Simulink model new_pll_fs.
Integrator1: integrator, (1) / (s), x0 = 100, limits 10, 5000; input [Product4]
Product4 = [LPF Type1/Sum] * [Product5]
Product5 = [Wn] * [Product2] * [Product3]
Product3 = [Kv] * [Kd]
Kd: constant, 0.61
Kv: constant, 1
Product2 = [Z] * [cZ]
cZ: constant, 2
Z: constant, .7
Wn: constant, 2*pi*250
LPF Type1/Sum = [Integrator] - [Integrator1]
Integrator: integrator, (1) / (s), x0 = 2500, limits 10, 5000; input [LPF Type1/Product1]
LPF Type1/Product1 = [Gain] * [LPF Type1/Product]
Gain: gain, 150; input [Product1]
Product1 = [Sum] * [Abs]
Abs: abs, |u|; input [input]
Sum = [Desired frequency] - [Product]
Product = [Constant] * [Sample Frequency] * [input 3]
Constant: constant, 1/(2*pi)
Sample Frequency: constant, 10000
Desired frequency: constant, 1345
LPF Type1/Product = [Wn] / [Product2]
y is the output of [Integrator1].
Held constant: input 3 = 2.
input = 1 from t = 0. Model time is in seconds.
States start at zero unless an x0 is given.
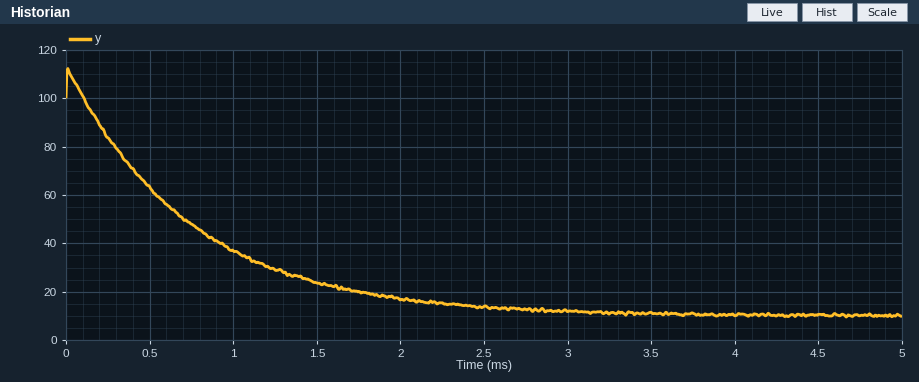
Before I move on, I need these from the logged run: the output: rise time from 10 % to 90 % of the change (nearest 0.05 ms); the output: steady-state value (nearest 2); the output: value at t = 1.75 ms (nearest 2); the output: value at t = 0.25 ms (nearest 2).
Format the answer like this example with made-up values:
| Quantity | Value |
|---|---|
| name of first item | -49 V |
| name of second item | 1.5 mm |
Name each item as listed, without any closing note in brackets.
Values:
| Quantity | Value |
|---|---|
| the output: rise time from 10 % to 90 % of the change | 1.65 ms |
| the output: steady-state value | 10 |
| the output: value at t = 1.75 ms | 20 |
| the output: value at t = 0.25 ms | 84 |
